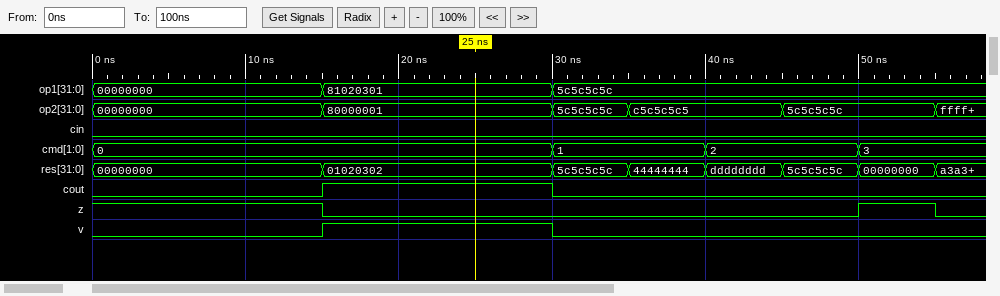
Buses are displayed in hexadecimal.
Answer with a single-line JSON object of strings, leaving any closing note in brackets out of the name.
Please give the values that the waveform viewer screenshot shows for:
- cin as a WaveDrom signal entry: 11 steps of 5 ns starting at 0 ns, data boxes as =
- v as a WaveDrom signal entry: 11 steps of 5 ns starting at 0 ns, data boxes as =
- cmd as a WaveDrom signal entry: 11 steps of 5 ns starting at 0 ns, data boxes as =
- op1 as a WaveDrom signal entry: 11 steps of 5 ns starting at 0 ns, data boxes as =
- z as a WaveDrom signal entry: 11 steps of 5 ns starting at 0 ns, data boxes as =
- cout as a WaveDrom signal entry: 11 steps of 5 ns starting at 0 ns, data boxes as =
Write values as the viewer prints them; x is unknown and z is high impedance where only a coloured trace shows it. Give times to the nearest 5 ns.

{"cin as a WaveDrom signal entry: 11 steps of 5 ns starting at 0 ns, data boxes as =": "{name: 'cin', wave: '0..........'}", "v as a WaveDrom signal entry: 11 steps of 5 ns starting at 0 ns, data boxes as =": "{name: 'v', wave: '0..1..0....'}", "cmd as a WaveDrom signal entry: 11 steps of 5 ns starting at 0 ns, data boxes as =": "{name: 'cmd', wave: '=.....=.=.=', data: '0 1 2 3'}", "op1 as a WaveDrom signal entry: 11 steps of 5 ns starting at 0 ns, data boxes as =": "{name: 'op1', wave: '=..=..=....', data: '00000000 81020301 5c5c5c5c'}", "z as a WaveDrom signal entry: 11 steps of 5 ns starting at 0 ns, data boxes as =": "{name: 'z', wave: '1..0......1'}", "cout as a WaveDrom signal entry: 11 steps of 5 ns starting at 0 ns, data boxes as =": "{name: 'cout', wave: '0..1..0....'}"}
